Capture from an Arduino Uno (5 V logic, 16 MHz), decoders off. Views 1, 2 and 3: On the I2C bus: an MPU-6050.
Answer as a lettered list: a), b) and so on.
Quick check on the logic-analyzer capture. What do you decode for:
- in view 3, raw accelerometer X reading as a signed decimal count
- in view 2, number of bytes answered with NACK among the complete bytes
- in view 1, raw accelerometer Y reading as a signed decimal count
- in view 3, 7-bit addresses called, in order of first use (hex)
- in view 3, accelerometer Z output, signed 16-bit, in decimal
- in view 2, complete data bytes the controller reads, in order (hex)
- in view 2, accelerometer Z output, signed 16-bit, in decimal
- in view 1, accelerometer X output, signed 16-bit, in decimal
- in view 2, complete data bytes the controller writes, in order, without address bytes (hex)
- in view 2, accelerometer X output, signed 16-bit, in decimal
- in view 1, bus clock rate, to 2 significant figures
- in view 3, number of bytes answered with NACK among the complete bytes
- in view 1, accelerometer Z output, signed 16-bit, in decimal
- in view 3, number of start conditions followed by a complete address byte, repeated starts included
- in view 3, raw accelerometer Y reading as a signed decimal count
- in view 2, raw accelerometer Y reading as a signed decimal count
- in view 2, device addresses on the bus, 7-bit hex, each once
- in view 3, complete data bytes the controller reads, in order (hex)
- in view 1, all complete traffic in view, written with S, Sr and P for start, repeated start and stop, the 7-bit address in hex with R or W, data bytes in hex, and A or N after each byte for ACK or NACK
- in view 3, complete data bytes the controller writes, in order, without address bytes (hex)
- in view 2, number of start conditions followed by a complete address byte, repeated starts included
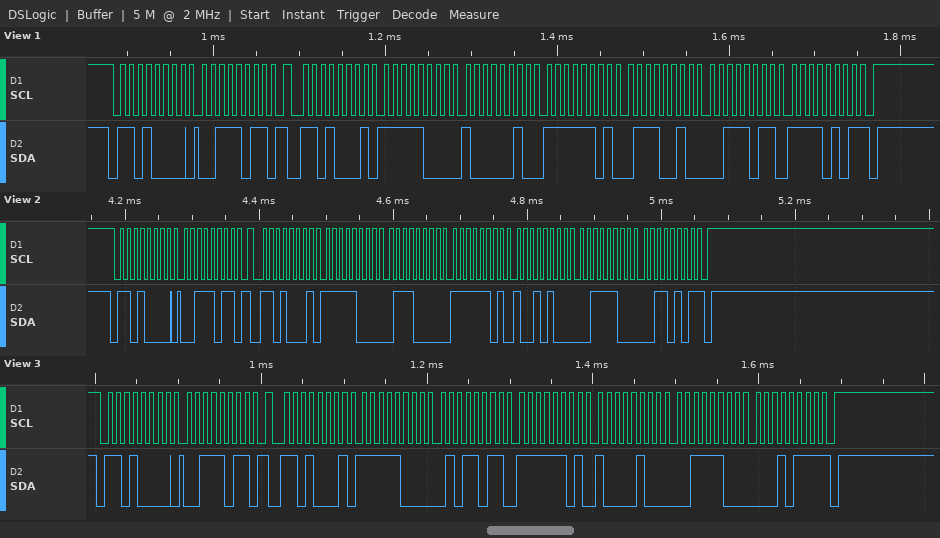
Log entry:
a) -1957
b) 1
c) -654
d) 0x68
e) 15383
f) F8 70 FD 94 3C 35
g) 15413
h) -1918
i) 3B
j) -1936
k) 100 kHz
l) 1
m) 15349
n) 2
o) -636
p) -620
q) 0x68
r) F8 5B FD 84 3C 17
s) S 68W A 3B A Sr 68R A F8 A 82 A FD A 72 A 3B A F5 N P
t) 3B
u) 2
